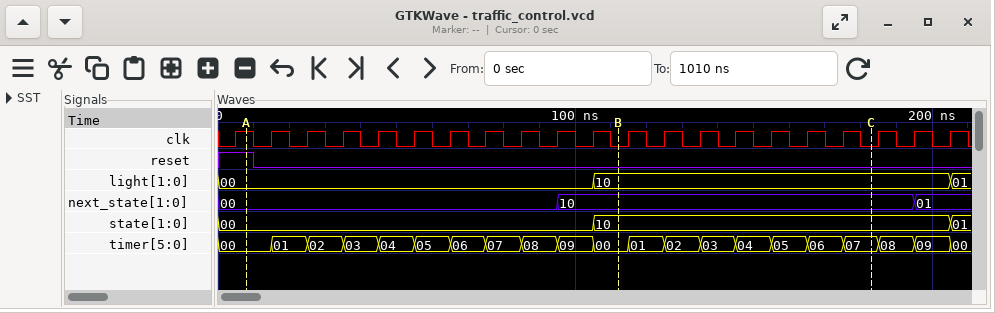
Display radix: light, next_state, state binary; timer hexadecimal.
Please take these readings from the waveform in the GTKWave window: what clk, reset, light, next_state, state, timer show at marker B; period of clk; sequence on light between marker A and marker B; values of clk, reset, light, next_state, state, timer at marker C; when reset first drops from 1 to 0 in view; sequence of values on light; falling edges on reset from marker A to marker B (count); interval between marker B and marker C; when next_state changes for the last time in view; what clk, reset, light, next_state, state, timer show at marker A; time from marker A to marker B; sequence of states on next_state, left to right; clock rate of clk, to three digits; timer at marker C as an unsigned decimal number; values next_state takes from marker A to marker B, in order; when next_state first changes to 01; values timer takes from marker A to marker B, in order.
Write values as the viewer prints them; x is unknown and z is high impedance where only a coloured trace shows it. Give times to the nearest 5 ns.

clk=0, reset=0, light=10, next_state=10, state=10, timer=00
10 ns
00, 10
clk=0, reset=0, light=10, next_state=10, state=10, timer=07
10 ns
00, 10, 01
1
70 ns
195 ns
clk=1, reset=1, light=00, next_state=00, state=00, timer=00
105 ns
00, 10, 01
100 MHz
7
00, 10
195 ns
00, 01, 02, 03, 04, 05, 06, 07, 08, 09, 00
